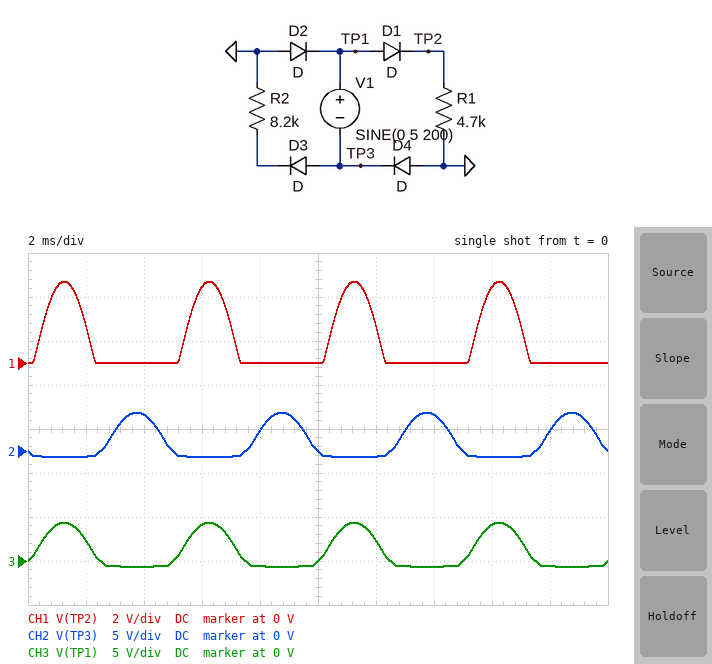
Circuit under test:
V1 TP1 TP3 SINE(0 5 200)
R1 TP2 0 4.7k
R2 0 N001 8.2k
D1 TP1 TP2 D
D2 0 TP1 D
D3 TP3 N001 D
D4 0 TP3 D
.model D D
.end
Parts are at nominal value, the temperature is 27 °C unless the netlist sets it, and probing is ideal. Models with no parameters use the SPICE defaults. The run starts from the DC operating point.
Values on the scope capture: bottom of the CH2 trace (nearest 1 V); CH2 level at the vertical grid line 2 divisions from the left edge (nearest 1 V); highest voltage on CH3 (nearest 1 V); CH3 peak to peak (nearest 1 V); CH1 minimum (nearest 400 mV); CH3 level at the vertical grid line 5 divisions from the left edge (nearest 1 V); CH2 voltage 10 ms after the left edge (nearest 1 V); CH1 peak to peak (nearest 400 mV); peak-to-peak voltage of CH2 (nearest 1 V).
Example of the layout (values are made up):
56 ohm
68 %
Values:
-1 V
4 V
4 V
5 V
0 V
0 V
0 V
3.6 V
5 V
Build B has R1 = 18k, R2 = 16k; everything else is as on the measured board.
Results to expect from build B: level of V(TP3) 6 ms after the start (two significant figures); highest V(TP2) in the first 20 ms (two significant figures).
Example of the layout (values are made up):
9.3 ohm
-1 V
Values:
-610 mV
3.8 V
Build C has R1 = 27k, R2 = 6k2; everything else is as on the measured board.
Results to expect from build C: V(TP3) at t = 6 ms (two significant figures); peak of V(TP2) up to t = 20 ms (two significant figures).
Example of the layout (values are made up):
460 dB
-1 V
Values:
-600 mV
3.8 V
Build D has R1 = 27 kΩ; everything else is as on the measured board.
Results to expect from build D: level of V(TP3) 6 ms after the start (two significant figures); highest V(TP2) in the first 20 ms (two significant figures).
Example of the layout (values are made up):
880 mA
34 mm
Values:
-600 mV
3.8 V
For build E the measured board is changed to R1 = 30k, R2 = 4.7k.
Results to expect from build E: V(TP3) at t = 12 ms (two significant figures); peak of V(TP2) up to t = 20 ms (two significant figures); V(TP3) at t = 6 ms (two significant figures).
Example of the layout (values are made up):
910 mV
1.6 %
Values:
-580 mV
3.8 V
-600 mV
